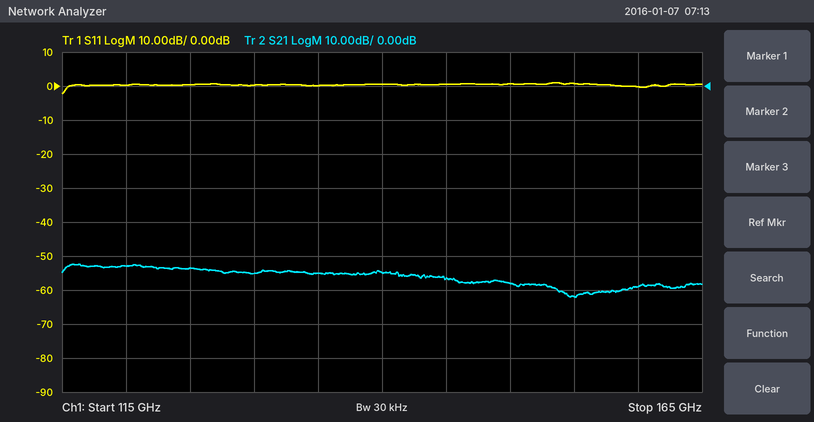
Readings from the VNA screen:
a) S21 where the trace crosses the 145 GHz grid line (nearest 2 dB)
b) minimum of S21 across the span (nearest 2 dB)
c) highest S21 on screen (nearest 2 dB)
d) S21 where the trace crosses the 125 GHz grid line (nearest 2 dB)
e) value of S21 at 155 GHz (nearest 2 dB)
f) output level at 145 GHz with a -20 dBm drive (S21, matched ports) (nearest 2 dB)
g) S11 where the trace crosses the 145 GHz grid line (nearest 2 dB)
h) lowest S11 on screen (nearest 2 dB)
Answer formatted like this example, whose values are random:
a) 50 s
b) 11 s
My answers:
a) -56 dB
b) -62 dB
c) -52 dB
d) -54 dB
e) -62 dB
f) -76 dBm
g) 0 dB
h) -2 dB
